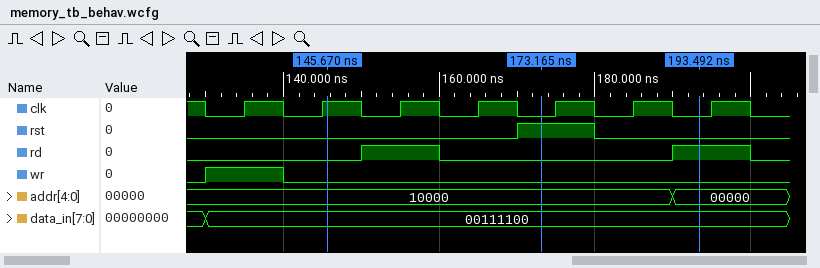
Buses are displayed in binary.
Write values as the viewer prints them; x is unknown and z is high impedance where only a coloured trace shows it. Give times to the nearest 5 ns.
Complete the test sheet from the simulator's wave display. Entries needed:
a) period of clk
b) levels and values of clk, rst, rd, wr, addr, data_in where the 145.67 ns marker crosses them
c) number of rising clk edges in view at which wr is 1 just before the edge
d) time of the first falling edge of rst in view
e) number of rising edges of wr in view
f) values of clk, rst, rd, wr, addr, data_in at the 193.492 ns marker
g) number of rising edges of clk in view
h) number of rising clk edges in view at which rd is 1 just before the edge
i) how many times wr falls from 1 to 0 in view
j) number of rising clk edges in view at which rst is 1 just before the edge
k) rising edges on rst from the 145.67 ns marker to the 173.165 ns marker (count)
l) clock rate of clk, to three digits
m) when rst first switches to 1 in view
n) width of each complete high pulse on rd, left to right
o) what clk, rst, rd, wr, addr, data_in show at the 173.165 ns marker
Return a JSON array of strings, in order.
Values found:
["10 ns", "clk=1, rst=0, rd=0, wr=0, addr=10000, data_in=00111100", "1", "180 ns", "1", "clk=0, rst=0, rd=1, wr=0, addr=00000, data_in=00111100", "7", "2", "1", "1", "1", "100 MHz", "170 ns", "10 ns, 10 ns", "clk=0, rst=1, rd=0, wr=0, addr=10000, data_in=00111100"]
